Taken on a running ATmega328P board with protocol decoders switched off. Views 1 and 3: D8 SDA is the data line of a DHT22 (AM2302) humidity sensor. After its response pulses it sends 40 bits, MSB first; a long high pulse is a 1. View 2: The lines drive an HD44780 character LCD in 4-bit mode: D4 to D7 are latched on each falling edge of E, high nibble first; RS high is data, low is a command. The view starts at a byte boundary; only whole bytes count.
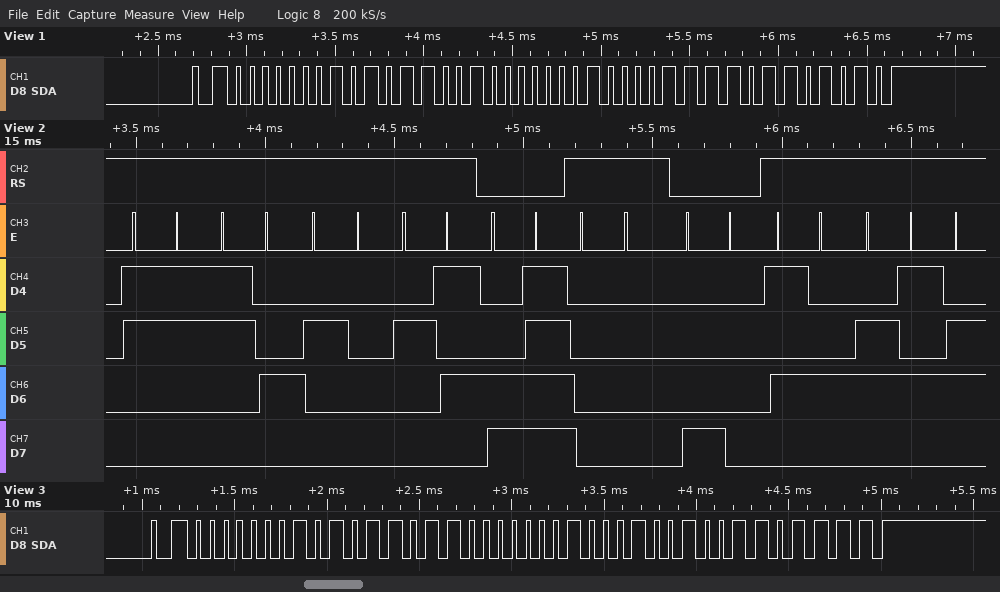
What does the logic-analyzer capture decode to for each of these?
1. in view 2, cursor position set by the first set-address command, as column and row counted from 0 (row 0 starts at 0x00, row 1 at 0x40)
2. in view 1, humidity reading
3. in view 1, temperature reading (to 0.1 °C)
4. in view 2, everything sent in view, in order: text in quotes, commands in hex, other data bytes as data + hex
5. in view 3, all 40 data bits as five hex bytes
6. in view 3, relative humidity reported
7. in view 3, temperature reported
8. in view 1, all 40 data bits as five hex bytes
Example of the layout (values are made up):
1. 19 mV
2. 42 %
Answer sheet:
1. column 15, row 1
2. 34.5 %
3. 27.1 °C
4. "34 %" 0xCF data 00 0x80 "Te"
5. 01 5B 01 12 6F
6. 34.7 %
7. 27.4 °C
8. 01 59 01 0F 6A
